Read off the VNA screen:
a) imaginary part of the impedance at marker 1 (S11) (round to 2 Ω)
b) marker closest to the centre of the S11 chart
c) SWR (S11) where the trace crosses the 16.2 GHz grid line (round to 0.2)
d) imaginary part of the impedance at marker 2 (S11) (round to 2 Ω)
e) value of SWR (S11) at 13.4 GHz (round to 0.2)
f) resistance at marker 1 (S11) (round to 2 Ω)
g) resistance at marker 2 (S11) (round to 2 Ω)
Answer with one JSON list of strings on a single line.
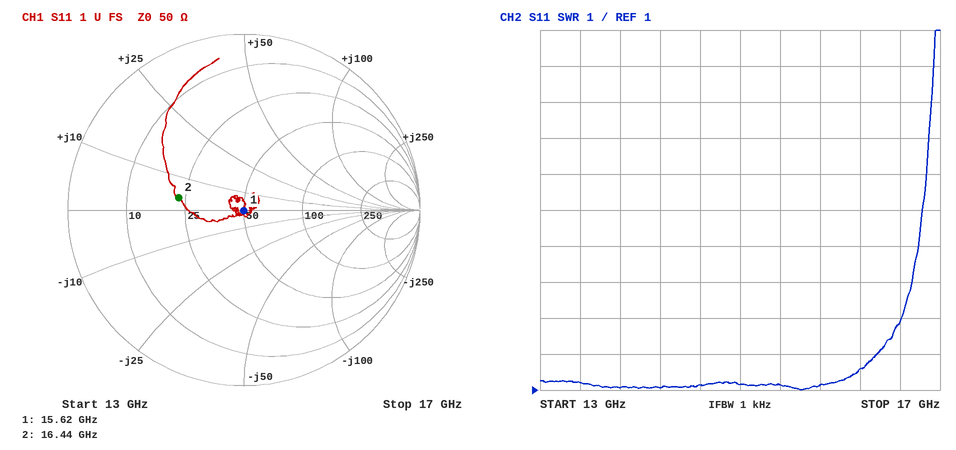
["0 Ω", "marker 1", "1.6", "+4 Ω", "1.2", "50 Ω", "22 Ω"]
